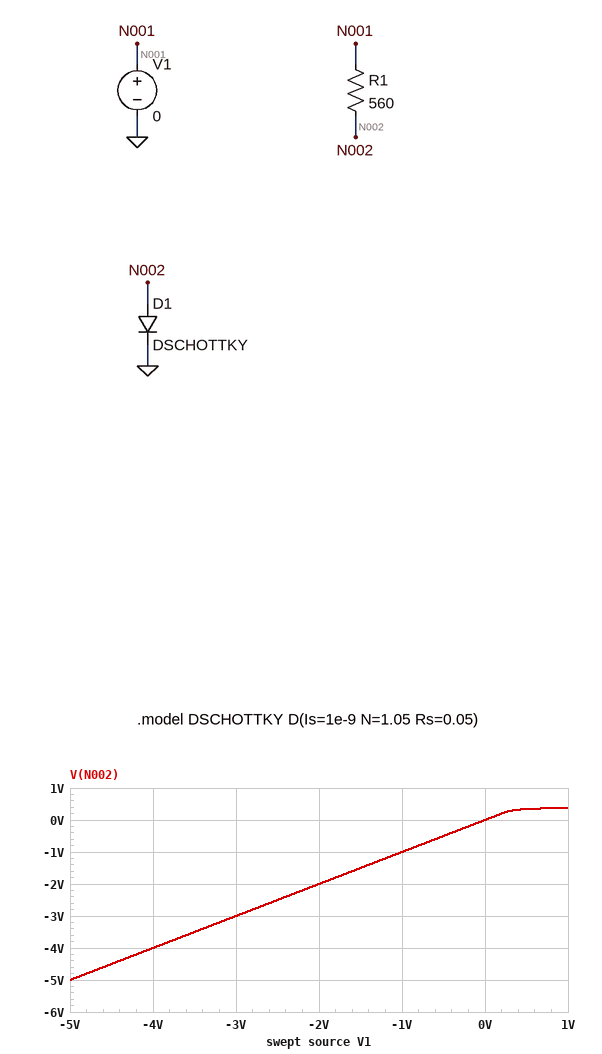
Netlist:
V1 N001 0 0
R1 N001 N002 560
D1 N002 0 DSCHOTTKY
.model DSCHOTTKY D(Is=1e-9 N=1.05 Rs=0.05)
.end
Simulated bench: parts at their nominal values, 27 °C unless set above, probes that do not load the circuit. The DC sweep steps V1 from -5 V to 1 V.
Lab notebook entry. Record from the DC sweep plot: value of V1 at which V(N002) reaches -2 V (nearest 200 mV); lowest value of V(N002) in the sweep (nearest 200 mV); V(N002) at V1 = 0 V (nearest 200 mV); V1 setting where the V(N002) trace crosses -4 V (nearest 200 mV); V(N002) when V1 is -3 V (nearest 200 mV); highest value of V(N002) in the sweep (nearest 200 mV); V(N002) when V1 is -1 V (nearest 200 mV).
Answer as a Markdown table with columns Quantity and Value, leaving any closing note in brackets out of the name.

| Quantity | Value |
|---|---|
| value of V1 at which V(N002) reaches -2 V | -2.0 V |
| lowest value of V(N002) in the sweep | -5.0 V |
| V(N002) at V1 = 0 V | 0 V |
| V1 setting where the V(N002) trace crosses -4 V | -4.0 V |
| V(N002) when V1 is -3 V | -3.0 V |
| highest value of V(N002) in the sweep | 400 mV |
| V(N002) when V1 is -1 V | -1.0 V |
